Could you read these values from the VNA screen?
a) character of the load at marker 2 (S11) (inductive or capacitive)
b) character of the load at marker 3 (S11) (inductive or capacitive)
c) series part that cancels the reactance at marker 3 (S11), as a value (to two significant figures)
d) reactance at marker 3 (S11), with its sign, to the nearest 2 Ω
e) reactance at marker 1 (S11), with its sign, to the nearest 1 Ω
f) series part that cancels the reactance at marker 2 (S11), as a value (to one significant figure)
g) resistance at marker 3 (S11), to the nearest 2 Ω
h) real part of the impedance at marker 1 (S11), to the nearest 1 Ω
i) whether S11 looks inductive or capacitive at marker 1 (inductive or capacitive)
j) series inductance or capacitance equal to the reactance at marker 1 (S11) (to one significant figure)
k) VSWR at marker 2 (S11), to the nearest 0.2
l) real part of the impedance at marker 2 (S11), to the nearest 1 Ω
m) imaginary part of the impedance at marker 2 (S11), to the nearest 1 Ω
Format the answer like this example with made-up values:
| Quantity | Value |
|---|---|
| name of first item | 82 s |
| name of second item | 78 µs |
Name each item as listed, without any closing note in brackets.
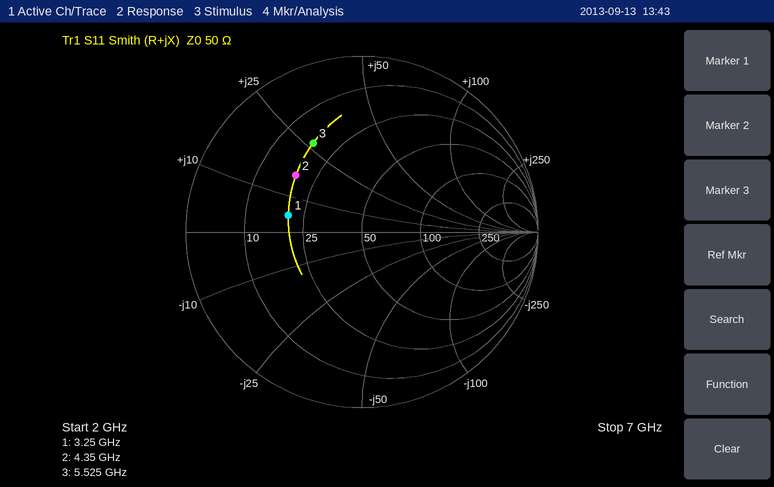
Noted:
| Quantity | Value |
|---|---|
| character of the load at marker 2 (S11) | inductive |
| character of the load at marker 3 (S11) | inductive |
| series part that cancels the reactance at marker 3 (S11), as a value | 1.1 pF |
| reactance at marker 3 (S11), with its sign, to the nearest 2 Ω | +26 Ω |
| reactance at marker 1 (S11), with its sign, to the nearest 1 Ω | +5 Ω |
| series part that cancels the reactance at marker 2 (S11), as a value | 2 pF |
| resistance at marker 3 (S11), to the nearest 2 Ω | 18 Ω |
| real part of the impedance at marker 1 (S11), to the nearest 1 Ω | 20 Ω |
| whether S11 looks inductive or capacitive at marker 1 | inductive |
| series inductance or capacitance equal to the reactance at marker 1 (S11) | 200 pH |
| VSWR at marker 2 (S11), to the nearest 0.2 | 3.0 |
| real part of the impedance at marker 2 (S11), to the nearest 1 Ω | 19 Ω |
| imaginary part of the impedance at marker 2 (S11), to the nearest 1 Ω | +16 Ω |
